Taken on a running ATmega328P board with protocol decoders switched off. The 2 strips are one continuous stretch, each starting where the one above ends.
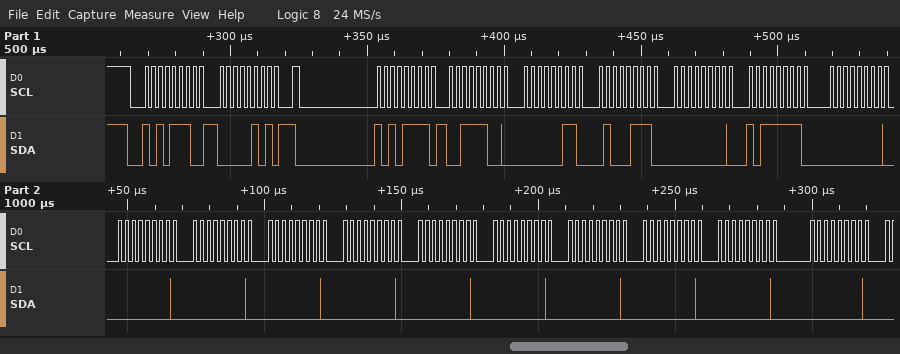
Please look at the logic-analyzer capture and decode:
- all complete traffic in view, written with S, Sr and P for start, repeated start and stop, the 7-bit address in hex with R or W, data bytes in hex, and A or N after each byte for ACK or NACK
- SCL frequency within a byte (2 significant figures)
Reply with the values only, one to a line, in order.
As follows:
S 57W A 05 A Sr 57R A 3C A 03 A 47 A 00 A BF A 00 A 00 A 00 A 00 A 00 A 00 A 00 A 00 A 00 A 00 A 00 A
400 kHz
